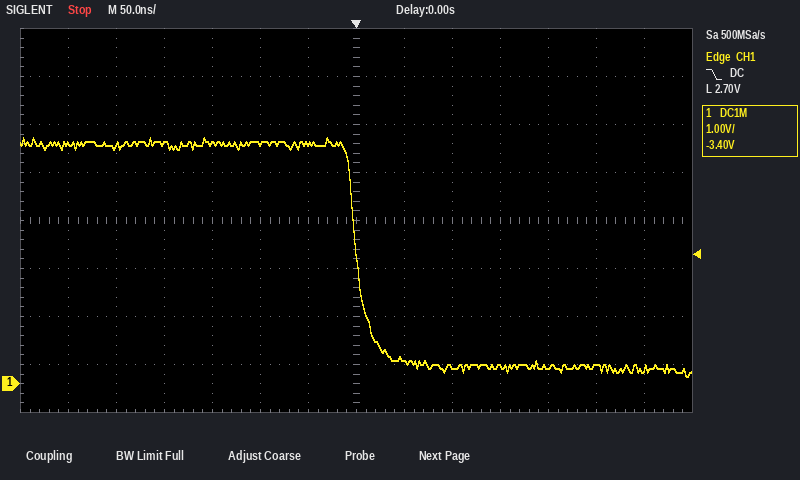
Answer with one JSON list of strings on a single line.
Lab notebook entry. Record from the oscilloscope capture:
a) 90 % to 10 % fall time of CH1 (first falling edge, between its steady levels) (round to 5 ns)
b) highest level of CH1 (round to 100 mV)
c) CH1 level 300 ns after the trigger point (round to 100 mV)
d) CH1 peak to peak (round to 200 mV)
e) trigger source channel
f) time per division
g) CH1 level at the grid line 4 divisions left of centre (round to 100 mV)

["30 ns", "5.1 V", "300 mV", "5.0 V", "CH1", "50 ns", "5.0 V"]
